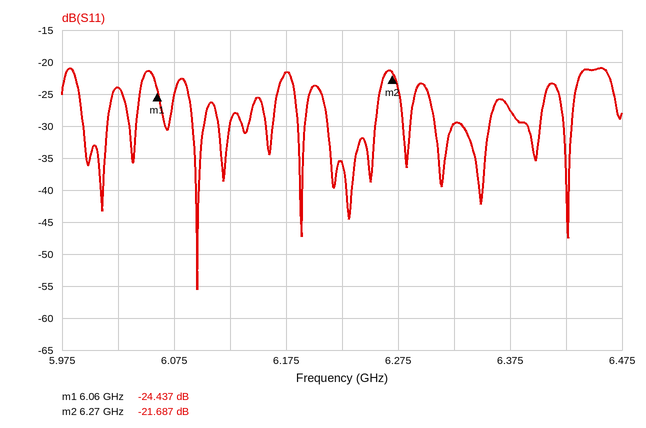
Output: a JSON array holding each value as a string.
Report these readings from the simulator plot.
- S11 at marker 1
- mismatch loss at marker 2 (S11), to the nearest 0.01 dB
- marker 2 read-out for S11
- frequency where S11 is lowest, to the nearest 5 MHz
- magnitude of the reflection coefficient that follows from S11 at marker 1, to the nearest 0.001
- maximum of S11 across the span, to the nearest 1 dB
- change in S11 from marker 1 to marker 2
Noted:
["-24.437 dB", "0.03 dB", "-21.687 dB", "6.095 GHz", "0.060", "-21 dB", "2.750 dB"]
